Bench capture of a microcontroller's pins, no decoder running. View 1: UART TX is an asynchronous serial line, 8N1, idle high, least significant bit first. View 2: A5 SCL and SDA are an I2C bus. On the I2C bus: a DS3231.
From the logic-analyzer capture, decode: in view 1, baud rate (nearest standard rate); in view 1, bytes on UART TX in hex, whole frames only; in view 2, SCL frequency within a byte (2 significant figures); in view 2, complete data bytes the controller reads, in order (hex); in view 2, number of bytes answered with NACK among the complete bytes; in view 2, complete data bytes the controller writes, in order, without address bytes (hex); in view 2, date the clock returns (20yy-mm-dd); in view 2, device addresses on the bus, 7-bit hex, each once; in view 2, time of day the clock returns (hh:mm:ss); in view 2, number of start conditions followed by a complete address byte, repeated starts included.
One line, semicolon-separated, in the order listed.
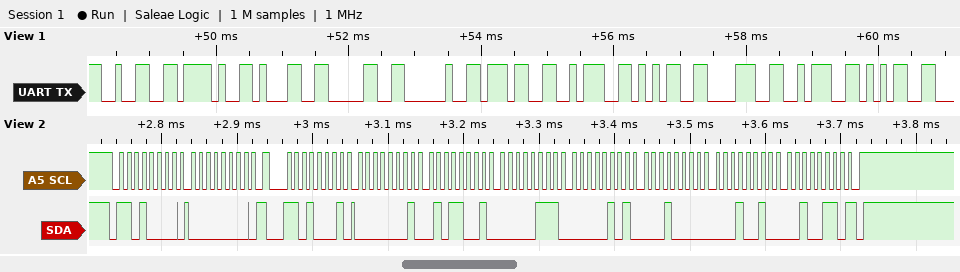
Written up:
9600 baud; 0x32 0x2F 0x31 0x30 0x20 0x37 0x3A 0x35 0x38 0x3A 0x35; 100 kHz; 01 59 07 05 10 12 26; 1; 00; 2026-12-10; 0x68; 07:59:01; 2
